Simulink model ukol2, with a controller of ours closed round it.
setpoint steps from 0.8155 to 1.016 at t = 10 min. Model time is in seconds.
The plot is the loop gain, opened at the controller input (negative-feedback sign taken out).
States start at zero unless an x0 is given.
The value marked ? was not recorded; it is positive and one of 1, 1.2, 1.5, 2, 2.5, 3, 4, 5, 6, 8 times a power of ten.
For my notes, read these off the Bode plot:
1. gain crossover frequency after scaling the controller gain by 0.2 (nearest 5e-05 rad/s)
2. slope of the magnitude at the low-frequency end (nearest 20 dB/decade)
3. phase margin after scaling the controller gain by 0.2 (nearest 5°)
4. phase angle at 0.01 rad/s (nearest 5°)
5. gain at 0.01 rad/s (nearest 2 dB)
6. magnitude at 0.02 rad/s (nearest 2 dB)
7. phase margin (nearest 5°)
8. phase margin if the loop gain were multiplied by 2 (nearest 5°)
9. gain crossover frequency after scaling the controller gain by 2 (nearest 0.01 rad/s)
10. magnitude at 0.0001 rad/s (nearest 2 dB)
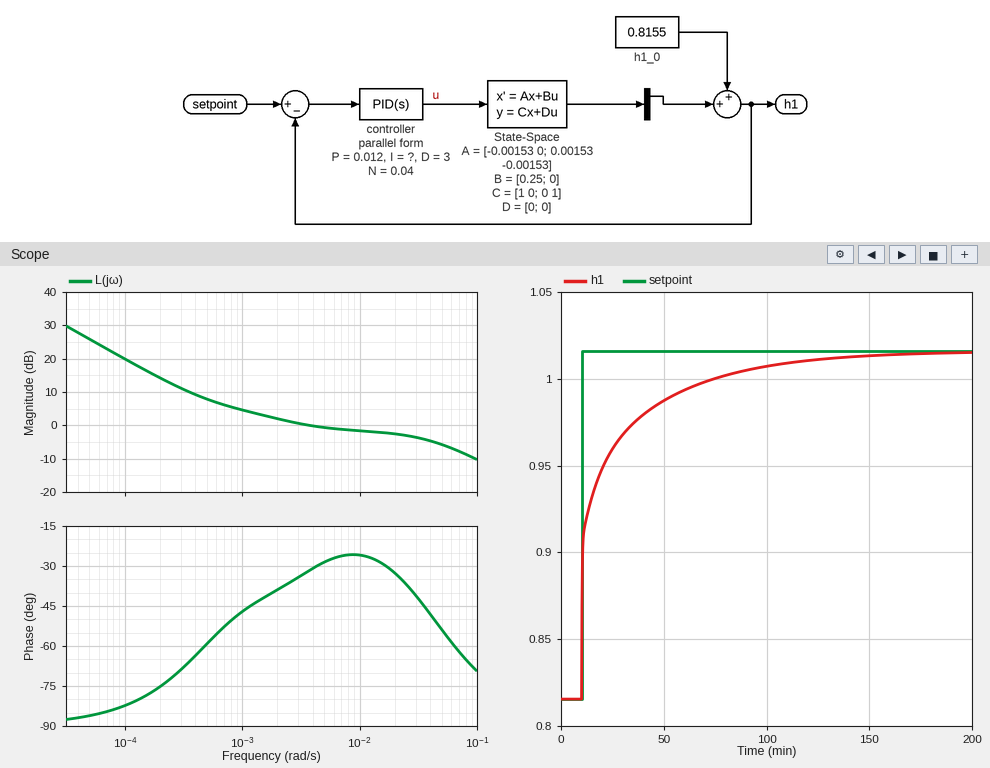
0.00020 rad/s
-20 dB/decade
105°
-25°
-2 dB
-2 dB
150°
125°
0.05 rad/s
20 dB
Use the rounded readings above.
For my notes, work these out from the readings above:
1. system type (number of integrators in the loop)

1
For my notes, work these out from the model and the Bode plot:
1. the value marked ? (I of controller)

6e-06
